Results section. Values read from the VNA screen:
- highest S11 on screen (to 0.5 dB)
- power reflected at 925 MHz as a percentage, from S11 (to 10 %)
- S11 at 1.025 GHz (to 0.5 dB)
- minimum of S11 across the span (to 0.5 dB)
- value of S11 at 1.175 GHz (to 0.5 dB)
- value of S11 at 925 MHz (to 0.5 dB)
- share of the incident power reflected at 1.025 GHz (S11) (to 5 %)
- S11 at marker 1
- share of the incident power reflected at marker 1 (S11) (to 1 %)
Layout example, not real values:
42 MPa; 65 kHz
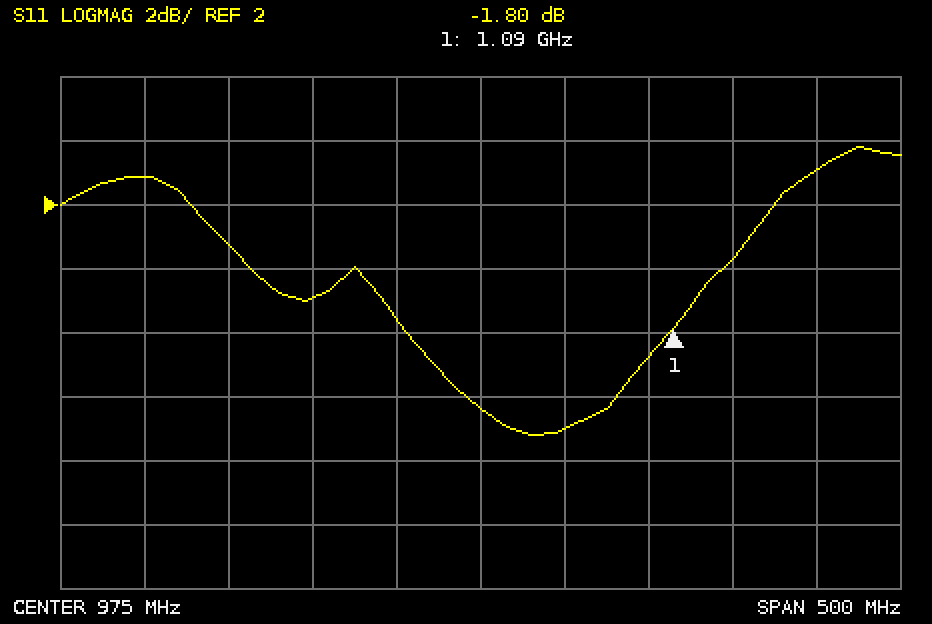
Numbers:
4.0 dB; 70 %; -5.0 dB; -5.0 dB; 3.0 dB; -1.5 dB; 30 %; -1.80 dB; 66 %
